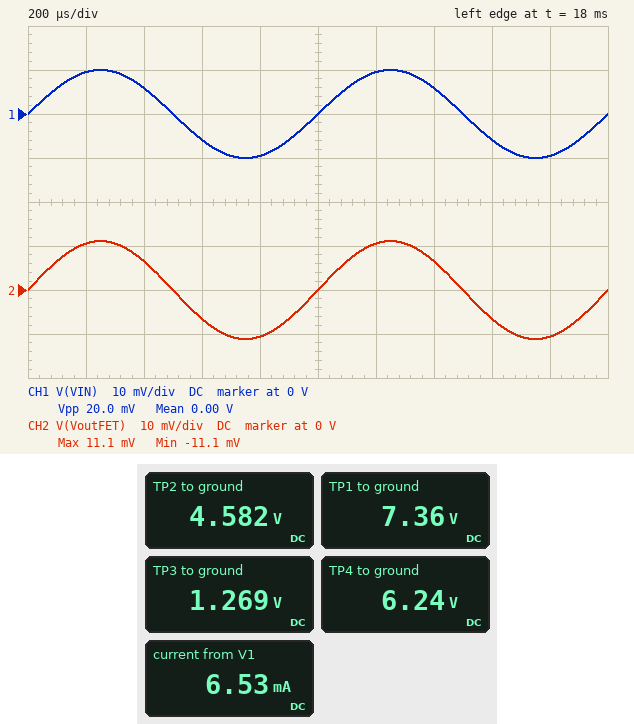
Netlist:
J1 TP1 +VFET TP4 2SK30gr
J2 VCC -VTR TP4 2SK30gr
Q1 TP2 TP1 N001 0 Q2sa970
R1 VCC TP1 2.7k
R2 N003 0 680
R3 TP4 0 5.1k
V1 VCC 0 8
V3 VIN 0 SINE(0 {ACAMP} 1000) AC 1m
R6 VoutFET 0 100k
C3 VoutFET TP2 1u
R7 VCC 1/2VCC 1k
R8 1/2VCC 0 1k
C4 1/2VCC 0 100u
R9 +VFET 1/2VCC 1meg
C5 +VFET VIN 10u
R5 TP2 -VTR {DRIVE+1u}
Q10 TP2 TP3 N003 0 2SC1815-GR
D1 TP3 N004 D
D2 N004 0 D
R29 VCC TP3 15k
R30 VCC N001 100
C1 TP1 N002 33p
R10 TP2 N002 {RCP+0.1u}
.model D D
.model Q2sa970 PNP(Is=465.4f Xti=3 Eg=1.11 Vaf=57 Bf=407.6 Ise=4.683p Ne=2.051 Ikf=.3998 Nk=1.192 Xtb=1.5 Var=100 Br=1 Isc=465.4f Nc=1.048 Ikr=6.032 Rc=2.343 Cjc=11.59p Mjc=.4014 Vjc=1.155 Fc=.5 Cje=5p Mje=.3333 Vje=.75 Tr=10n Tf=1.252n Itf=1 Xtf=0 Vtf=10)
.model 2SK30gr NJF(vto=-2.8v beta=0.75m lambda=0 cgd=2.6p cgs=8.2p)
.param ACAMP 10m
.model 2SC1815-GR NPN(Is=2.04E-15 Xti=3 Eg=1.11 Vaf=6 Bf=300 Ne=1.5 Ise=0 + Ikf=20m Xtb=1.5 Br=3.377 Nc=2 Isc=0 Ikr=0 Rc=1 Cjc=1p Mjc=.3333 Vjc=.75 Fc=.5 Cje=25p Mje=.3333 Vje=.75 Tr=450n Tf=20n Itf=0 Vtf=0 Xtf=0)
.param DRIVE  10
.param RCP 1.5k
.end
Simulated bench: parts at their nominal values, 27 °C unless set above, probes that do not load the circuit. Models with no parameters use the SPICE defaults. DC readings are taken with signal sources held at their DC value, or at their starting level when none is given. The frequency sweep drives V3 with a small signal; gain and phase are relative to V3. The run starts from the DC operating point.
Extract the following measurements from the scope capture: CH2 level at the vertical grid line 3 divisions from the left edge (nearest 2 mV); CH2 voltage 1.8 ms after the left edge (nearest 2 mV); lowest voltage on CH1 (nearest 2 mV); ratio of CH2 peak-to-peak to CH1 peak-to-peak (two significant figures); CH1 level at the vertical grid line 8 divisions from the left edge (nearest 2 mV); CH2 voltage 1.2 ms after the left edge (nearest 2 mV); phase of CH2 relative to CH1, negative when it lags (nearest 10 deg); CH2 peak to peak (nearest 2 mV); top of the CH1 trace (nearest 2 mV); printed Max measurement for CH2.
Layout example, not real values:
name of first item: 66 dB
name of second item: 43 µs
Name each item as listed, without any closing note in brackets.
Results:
CH2 level at the vertical grid line 3 divisions from the left edge: -6 mV
CH2 voltage 1.8 ms after the left edge: -10 mV
lowest voltage on CH1: -10 mV
ratio of CH2 peak-to-peak to CH1 peak-to-peak: 1.1
CH1 level at the vertical grid line 8 divisions from the left edge: -6 mV
CH2 voltage 1.2 ms after the left edge: 10 mV
phase of CH2 relative to CH1, negative when it lags: 0 deg
CH2 peak to peak: 22 mV
top of the CH1 trace: 10 mV
printed Max measurement for CH2: 11.1 mV
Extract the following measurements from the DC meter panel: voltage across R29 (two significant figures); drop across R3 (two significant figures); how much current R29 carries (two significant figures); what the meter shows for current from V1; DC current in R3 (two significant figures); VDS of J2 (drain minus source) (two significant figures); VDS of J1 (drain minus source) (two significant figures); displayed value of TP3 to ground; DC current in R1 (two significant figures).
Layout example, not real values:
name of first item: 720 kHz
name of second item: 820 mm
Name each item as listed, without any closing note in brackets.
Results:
voltage across R29: 6.7 V
drop across R3: 6.2 V
how much current R29 carries: 450 µA
what the meter shows for current from V1: 6.53 mA
DC current in R3: 1.2 mA
VDS of J2 (drain minus source): 1.8 V
VDS of J1 (drain minus source): 1.1 V
displayed value of TP3 to ground: 1.269 V
DC current in R1: 240 µA
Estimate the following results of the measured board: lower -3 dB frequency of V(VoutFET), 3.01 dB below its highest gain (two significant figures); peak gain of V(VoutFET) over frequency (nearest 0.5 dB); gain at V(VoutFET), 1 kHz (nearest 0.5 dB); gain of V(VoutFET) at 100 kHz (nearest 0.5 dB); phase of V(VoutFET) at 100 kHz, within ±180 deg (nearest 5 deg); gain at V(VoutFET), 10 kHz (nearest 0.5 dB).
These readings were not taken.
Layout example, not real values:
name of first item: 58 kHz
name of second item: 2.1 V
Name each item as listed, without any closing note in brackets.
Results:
lower -3 dB frequency of V(VoutFET), 3.01 dB below its highest gain: 1.6 Hz
peak gain of V(VoutFET) over frequency: 1.0 dB
gain at V(VoutFET), 1 kHz: 1.0 dB
gain of V(VoutFET) at 100 kHz: 1.0 dB
phase of V(VoutFET) at 100 kHz, within ±180 deg: -5 deg
gain at V(VoutFET), 10 kHz: 1.0 dB
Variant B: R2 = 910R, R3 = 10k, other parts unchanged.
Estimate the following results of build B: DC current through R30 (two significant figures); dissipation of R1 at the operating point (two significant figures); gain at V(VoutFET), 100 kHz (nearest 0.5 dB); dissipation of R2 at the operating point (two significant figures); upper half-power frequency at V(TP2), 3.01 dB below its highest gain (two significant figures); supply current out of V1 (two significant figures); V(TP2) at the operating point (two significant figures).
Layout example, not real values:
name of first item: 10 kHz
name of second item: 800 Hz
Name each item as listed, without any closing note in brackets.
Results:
DC current through R30: 650 µA
dissipation of R1 at the operating point: 140 µW
gain at V(VoutFET), 100 kHz: 0.5 dB
dissipation of R2 at the operating point: 390 µW
upper half-power frequency at V(TP2), 3.01 dB below its highest gain: 1.4 MHz
supply current out of V1: 5.7 mA
V(TP2) at the operating point: 4.2 V
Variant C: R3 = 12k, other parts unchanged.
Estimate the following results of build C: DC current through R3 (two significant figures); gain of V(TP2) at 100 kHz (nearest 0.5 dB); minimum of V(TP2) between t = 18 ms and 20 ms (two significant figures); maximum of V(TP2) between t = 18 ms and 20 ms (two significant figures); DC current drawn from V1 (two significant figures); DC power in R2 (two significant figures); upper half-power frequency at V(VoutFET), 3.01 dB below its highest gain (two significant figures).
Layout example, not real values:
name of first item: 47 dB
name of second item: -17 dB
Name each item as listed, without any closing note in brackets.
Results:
DC current through R3: 520 µA
gain of V(TP2) at 100 kHz: 0.5 dB
minimum of V(TP2) between t = 18 ms and 20 ms: 4.0 V
maximum of V(TP2) between t = 18 ms and 20 ms: 4.1 V
DC current drawn from V1: 5.8 mA
DC power in R2: 500 µW
upper half-power frequency at V(VoutFET), 3.01 dB below its highest gain: 1.3 MHz
